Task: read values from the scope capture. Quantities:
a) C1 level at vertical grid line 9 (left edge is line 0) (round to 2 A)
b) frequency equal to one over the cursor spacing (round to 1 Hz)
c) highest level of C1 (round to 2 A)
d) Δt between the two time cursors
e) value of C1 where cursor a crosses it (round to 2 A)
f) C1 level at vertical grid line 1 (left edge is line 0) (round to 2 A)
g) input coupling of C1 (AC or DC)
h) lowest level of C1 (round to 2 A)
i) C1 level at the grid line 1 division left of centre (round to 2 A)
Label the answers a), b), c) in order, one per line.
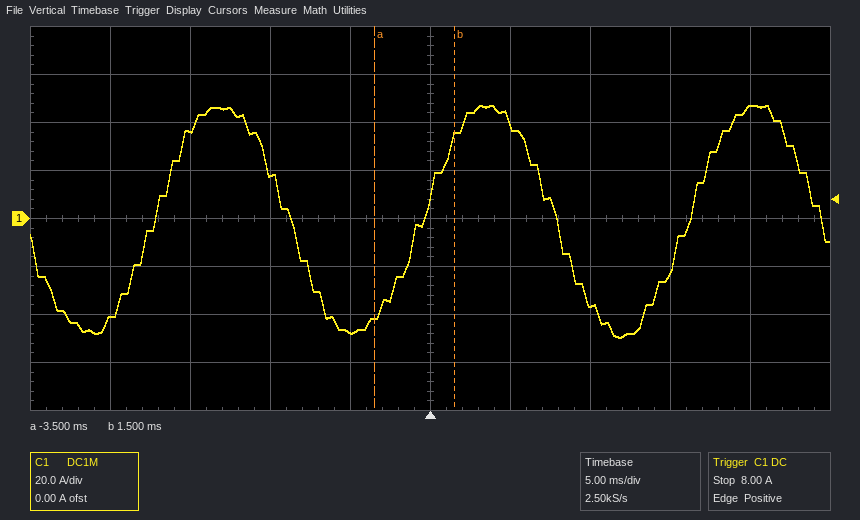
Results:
a) 46 A
b) 200 Hz
c) 48 A
d) 5.0 ms
e) -42 A
f) -42 A
g) DC
h) -50 A
i) -48 A
